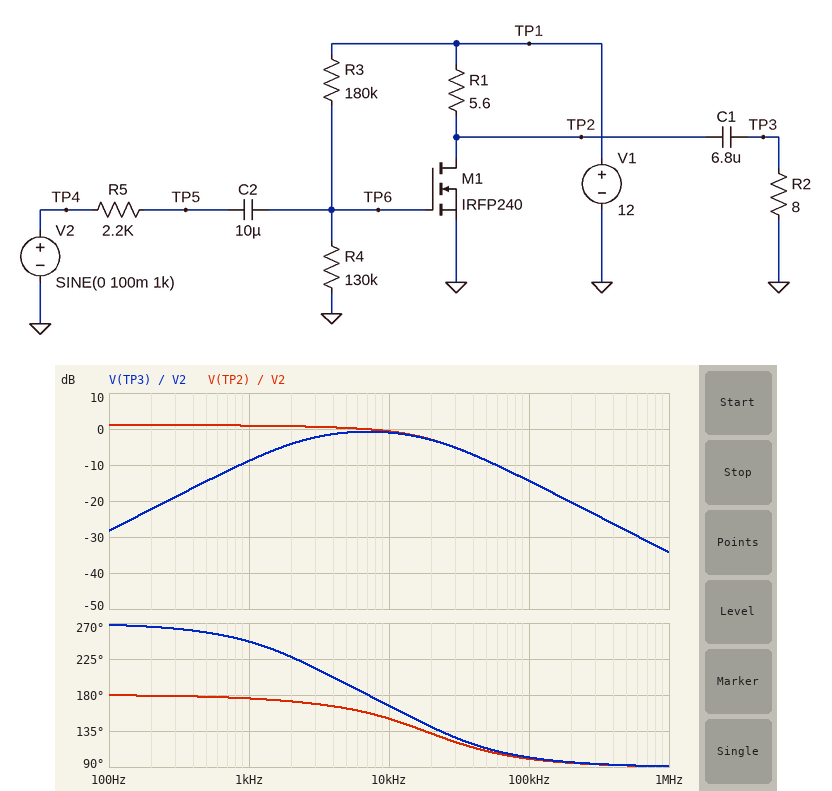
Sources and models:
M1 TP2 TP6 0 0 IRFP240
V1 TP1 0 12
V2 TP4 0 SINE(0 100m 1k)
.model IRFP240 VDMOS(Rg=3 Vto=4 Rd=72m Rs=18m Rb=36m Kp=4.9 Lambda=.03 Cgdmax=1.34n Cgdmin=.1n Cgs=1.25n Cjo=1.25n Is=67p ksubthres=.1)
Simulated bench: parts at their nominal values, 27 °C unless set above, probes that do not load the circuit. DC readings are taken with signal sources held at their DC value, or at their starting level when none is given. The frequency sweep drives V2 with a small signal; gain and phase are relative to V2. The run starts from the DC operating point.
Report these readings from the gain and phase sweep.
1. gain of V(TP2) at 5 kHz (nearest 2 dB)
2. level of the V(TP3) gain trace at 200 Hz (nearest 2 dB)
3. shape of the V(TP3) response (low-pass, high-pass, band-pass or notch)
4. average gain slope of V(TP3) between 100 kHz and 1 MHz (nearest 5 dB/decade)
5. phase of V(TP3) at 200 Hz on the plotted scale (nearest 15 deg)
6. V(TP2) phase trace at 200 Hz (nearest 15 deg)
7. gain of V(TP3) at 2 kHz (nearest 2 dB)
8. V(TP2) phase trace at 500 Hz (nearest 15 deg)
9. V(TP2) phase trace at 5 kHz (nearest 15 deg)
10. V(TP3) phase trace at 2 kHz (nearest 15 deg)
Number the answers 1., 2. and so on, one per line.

1. 0 dB
2. -22 dB
3. band-pass
4. -20 dB/decade
5. 270 deg
6. 180 deg
7. -4 dB
8. 180 deg
9. 165 deg
10. 225 deg
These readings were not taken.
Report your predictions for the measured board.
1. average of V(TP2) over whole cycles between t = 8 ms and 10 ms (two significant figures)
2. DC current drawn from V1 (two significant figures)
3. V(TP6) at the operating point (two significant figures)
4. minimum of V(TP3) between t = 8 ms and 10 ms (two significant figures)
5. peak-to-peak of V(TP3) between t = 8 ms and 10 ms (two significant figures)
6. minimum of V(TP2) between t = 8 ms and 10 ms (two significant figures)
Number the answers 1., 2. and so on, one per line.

1. 770 mV
2. 2.0 A
3. 5.0 V
4. -46 mV
5. 92 mV
6. 660 mV
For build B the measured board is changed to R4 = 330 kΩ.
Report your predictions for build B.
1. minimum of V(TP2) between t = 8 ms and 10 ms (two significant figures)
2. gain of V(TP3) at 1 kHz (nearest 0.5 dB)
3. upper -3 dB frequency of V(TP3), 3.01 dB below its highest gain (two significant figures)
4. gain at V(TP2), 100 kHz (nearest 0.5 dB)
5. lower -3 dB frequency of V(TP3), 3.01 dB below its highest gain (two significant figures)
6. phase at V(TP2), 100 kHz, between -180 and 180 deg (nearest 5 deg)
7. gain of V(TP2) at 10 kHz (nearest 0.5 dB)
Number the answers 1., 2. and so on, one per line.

1. 300 mV
2. -40.0 dB
3. 33 kHz
4. -42.0 dB
5. 2.4 kHz
6. 105 deg
7. -31.0 dB
